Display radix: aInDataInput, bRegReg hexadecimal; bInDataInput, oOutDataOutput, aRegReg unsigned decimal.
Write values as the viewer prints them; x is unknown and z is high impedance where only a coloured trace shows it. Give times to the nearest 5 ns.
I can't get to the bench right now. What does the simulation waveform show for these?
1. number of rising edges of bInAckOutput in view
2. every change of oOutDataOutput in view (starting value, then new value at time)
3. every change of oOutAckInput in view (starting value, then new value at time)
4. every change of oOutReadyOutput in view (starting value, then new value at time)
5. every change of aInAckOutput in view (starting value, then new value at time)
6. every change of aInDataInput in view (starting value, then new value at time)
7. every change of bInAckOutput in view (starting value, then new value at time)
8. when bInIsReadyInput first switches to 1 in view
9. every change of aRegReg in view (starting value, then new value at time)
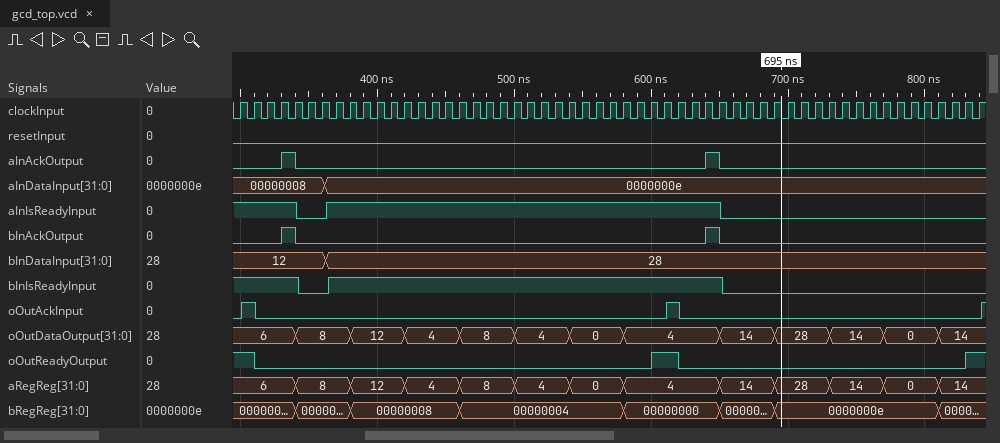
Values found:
2
6, 8 at 340 ns, 12 at 380 ns, 4 at 420 ns, 8 at 460 ns, 4 at 500 ns, 0 at 540 ns, 4 at 580 ns, 14 at 650 ns, 28 at 690 ns, 14 at 730 ns, 0 at 770 ns, 14 at 810 ns
0, 1 at 300 ns, 0 at 310 ns, 1 at 610 ns, 0 at 620 ns, 1 at 840 ns
1, 0 at 310 ns, 1 at 600 ns, 0 at 620 ns, 1 at 830 ns
0, 1 at 330 ns, 0 at 340 ns, 1 at 640 ns, 0 at 650 ns
00000008, 0000000e at 360 ns
0, 1 at 330 ns, 0 at 340 ns, 1 at 640 ns, 0 at 650 ns
365 ns
6, 8 at 340 ns, 12 at 380 ns, 4 at 420 ns, 8 at 460 ns, 4 at 500 ns, 0 at 540 ns, 4 at 580 ns, 14 at 650 ns, 28 at 690 ns, 14 at 730 ns, 0 at 770 ns, 14 at 810 ns
